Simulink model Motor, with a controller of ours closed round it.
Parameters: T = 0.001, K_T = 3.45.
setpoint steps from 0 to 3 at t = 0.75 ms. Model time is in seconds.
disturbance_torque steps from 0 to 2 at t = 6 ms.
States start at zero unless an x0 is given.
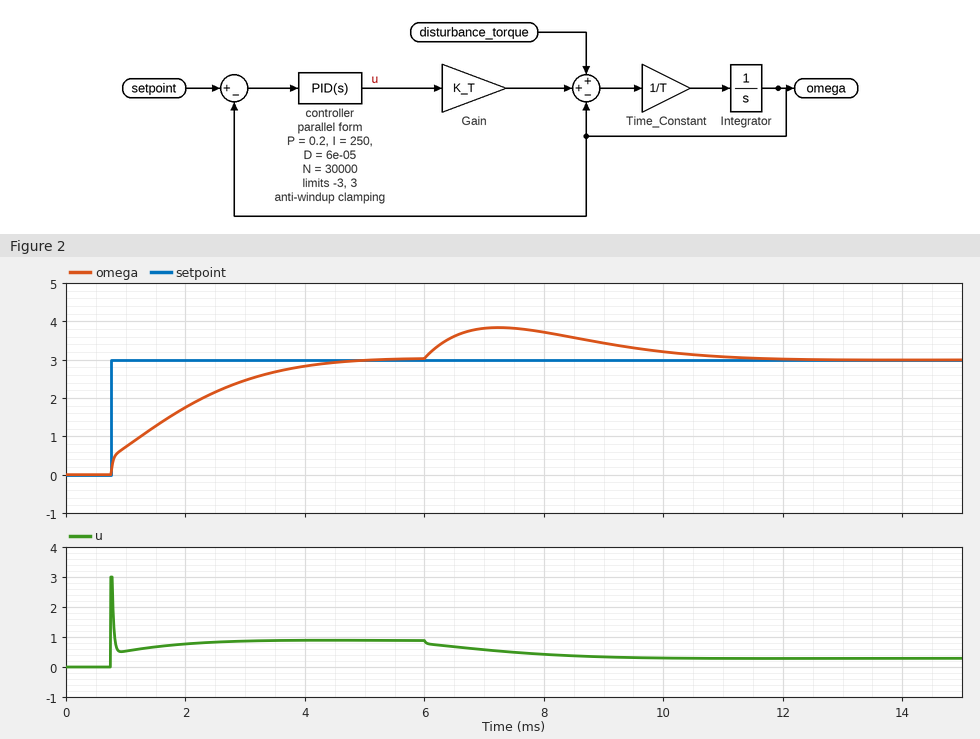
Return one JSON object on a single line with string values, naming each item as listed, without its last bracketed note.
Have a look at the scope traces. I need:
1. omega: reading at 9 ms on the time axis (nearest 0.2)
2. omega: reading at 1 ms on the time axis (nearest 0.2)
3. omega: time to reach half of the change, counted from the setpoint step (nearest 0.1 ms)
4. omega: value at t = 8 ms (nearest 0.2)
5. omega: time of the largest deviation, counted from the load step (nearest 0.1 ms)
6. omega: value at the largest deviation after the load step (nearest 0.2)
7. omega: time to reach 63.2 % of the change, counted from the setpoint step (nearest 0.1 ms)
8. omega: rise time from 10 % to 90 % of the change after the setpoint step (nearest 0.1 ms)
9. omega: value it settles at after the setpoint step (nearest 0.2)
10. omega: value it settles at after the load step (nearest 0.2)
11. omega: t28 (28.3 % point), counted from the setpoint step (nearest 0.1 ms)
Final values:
{"omega: reading at 9 ms on the time axis": "3.4", "omega: reading at 1 ms on the time axis": "0.8", "omega: time to reach half of the change, counted from the setpoint step": "1.0 ms", "omega: value at t = 8 ms": "3.8", "omega: time of the largest deviation, counted from the load step": "1.2 ms", "omega: value at the largest deviation after the load step": "3.8", "omega: time to reach 63.2 % of the change, counted from the setpoint step": "1.4 ms", "omega: rise time from 10 % to 90 % of the change after the setpoint step": "2.8 ms", "omega: value it settles at after the setpoint step": "3.0", "omega: value it settles at after the load step": "3.0", "omega: t28 (28.3 % point), counted from the setpoint step": "0.4 ms"}
